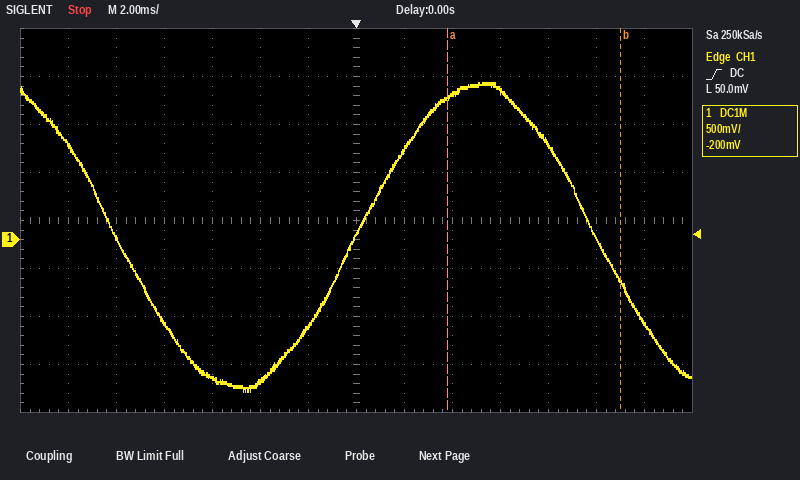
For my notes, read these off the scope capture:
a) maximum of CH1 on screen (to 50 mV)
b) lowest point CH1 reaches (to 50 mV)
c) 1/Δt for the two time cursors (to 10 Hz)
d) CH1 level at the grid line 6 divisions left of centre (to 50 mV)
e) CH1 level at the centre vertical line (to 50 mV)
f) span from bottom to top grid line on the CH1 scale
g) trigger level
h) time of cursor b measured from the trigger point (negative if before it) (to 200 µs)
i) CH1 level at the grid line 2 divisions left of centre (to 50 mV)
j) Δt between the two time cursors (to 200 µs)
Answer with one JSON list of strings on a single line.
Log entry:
["1.65 V", "-1.60 V", "140 Hz", "1.00 V", "50 mV", "4 V", "50.0 mV", "+11.0 ms", "-1.45 V", "7.2 ms"]
